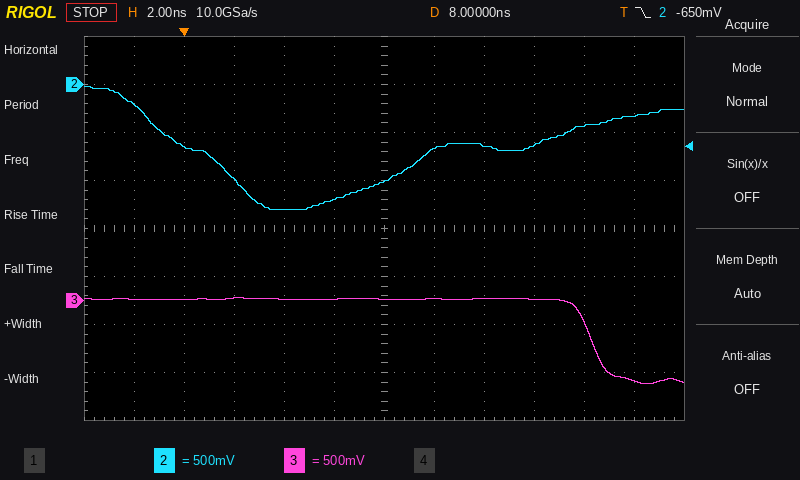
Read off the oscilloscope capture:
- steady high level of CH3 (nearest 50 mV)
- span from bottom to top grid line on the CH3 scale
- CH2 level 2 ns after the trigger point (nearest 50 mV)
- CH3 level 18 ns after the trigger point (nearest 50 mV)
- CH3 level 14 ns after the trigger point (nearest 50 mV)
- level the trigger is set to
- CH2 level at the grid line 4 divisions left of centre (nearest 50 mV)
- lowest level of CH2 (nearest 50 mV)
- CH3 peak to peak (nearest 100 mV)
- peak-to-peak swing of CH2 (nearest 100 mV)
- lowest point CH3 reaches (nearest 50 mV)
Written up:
0 mV
4 V
-1.00 V
-850 mV
0 mV
-650 mV
-650 mV
-1.30 V
900 mV
1.30 V
-850 mV
